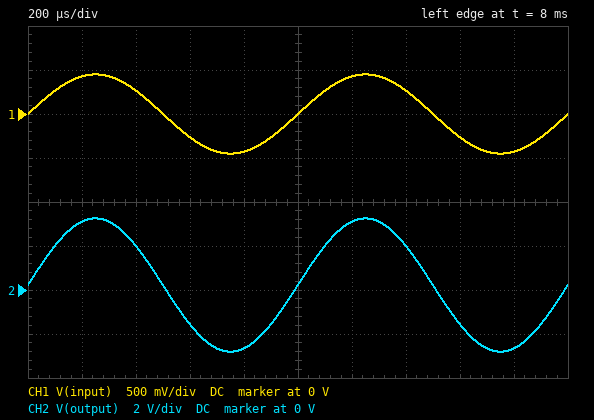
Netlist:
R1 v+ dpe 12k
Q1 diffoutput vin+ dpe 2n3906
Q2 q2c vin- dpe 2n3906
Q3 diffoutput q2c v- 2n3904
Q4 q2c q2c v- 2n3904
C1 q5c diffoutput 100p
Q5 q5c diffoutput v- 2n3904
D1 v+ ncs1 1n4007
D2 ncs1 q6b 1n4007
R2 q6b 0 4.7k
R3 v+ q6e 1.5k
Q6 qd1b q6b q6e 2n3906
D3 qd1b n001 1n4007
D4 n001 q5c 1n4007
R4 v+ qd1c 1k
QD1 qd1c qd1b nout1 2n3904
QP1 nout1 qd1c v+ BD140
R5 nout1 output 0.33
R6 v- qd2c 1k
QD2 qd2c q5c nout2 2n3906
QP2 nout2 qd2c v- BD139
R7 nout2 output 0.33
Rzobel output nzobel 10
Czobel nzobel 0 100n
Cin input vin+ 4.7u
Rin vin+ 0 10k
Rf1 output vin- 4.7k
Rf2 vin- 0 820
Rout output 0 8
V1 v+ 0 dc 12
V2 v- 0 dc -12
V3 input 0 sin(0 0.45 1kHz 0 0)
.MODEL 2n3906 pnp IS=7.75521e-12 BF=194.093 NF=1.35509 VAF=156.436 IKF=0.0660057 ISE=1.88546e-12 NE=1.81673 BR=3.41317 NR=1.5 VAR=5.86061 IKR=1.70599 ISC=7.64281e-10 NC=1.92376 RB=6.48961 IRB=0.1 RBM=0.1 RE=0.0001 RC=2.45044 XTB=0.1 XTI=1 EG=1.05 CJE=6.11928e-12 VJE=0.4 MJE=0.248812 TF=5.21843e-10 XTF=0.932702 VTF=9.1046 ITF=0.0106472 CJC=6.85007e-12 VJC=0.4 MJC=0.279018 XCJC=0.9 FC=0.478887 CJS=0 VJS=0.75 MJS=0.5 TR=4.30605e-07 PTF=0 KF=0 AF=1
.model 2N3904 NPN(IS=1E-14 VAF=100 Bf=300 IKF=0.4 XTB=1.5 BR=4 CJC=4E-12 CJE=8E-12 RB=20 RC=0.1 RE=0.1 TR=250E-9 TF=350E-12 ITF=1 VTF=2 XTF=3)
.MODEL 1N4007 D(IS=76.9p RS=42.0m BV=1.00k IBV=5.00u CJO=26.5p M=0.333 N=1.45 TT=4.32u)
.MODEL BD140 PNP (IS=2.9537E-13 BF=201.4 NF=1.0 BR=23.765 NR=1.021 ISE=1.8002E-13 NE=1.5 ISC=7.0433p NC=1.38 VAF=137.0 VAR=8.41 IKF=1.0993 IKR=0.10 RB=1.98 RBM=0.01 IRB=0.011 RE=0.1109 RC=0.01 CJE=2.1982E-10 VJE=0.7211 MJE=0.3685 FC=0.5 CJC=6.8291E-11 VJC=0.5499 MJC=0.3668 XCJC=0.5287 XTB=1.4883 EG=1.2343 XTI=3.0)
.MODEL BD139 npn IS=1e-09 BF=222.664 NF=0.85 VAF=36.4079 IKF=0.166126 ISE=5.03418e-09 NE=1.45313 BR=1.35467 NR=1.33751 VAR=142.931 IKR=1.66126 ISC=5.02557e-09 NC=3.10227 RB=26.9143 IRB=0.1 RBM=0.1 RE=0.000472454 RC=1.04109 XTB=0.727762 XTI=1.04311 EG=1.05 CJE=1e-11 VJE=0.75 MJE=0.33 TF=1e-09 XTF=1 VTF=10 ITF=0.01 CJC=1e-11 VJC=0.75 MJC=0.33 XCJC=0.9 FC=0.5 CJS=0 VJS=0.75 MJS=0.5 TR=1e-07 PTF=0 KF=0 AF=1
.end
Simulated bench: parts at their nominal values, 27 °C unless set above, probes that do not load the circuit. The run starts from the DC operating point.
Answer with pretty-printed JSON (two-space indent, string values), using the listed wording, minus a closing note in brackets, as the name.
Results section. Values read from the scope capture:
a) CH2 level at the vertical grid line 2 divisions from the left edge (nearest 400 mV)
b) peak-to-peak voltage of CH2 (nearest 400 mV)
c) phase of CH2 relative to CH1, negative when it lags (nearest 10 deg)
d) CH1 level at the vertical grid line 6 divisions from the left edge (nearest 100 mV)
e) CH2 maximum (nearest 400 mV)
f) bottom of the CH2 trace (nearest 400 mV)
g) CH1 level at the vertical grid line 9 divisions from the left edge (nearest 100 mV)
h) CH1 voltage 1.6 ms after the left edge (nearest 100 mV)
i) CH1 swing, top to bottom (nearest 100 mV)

{
  "CH2 level at the vertical grid line 2 divisions from the left edge": "2.0 V",
  "peak-to-peak voltage of CH2": "6.0 V",
  "phase of CH2 relative to CH1, negative when it lags": "0 deg",
  "CH1 level at the vertical grid line 6 divisions from the left edge": "400 mV",
  "CH2 maximum": "3.2 V",
  "bottom of the CH2 trace": "-2.8 V",
  "CH1 level at the vertical grid line 9 divisions from the left edge": "-400 mV",
  "CH1 voltage 1.6 ms after the left edge": "-300 mV",
  "CH1 swing, top to bottom": "900 mV"
}
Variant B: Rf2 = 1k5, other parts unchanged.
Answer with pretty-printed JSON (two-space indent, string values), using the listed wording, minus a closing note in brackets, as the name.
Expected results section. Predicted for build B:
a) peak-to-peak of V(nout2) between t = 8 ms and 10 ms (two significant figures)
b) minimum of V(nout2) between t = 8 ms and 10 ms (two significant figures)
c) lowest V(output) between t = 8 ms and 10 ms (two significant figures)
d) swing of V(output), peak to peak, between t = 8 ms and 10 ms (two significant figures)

{
  "peak-to-peak of V(nout2) between t = 8 ms and 10 ms": "3.8 V",
  "minimum of V(nout2) between t = 8 ms and 10 ms": "-1.8 V",
  "lowest V(output) between t = 8 ms and 10 ms": "-1.7 V",
  "swing of V(output), peak to peak, between t = 8 ms and 10 ms": "3.7 V"
}
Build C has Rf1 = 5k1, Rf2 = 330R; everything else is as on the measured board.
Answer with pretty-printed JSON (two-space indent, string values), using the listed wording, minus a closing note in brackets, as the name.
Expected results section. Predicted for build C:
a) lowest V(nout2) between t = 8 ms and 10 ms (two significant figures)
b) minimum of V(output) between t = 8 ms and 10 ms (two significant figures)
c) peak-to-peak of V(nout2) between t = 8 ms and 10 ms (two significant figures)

{
  "lowest V(nout2) between t = 8 ms and 10 ms": "-7.1 V",
  "minimum of V(output) between t = 8 ms and 10 ms": "-6.8 V",
  "peak-to-peak of V(nout2) between t = 8 ms and 10 ms": "15 V"
}
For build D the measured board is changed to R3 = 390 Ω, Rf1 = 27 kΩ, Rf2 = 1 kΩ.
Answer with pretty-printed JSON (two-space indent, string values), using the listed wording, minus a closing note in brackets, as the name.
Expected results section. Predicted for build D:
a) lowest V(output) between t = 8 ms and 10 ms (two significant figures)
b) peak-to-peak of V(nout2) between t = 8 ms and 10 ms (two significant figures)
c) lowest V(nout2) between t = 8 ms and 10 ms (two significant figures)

{
  "lowest V(output) between t = 8 ms and 10 ms": "-10 V",
  "peak-to-peak of V(nout2) between t = 8 ms and 10 ms": "21 V",
  "lowest V(nout2) between t = 8 ms and 10 ms": "-11 V"
}
